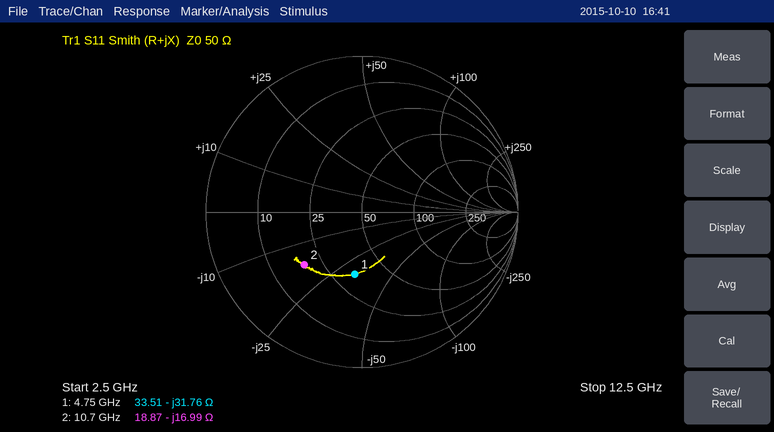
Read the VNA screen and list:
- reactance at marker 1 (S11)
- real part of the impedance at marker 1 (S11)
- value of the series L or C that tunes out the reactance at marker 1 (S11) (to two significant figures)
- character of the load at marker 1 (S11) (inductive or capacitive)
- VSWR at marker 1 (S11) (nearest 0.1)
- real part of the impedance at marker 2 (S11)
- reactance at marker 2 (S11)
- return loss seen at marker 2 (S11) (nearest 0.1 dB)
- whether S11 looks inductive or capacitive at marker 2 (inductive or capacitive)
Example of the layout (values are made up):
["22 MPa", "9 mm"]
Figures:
["-31.76 Ω", "33.51 Ω", "1.1 nH", "capacitive", "2.3", "18.87 Ω", "-16.99 Ω", "6.0 dB", "capacitive"]
